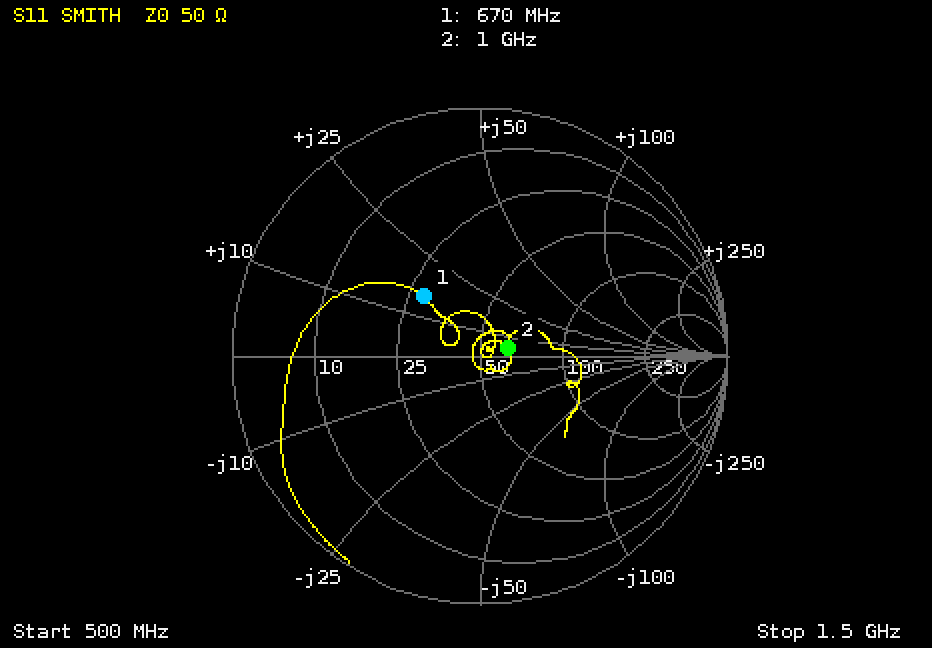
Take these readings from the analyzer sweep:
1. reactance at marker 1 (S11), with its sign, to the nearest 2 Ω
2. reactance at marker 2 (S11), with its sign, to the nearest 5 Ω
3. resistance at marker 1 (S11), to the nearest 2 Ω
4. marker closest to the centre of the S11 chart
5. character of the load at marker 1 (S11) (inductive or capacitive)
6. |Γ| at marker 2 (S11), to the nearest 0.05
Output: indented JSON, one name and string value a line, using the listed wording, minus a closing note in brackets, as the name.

{
  "reactance at marker 1 (S11), with its sign, to the nearest 2 Ω": "+16 Ω",
  "reactance at marker 2 (S11), with its sign, to the nearest 5 Ω": "+5 Ω",
  "resistance at marker 1 (S11), to the nearest 2 Ω": "28 Ω",
  "marker closest to the centre of the S11 chart": "marker 2",
  "character of the load at marker 1 (S11)": "inductive",
  "|Γ| at marker 2 (S11), to the nearest 0.05": "0.10"
}
